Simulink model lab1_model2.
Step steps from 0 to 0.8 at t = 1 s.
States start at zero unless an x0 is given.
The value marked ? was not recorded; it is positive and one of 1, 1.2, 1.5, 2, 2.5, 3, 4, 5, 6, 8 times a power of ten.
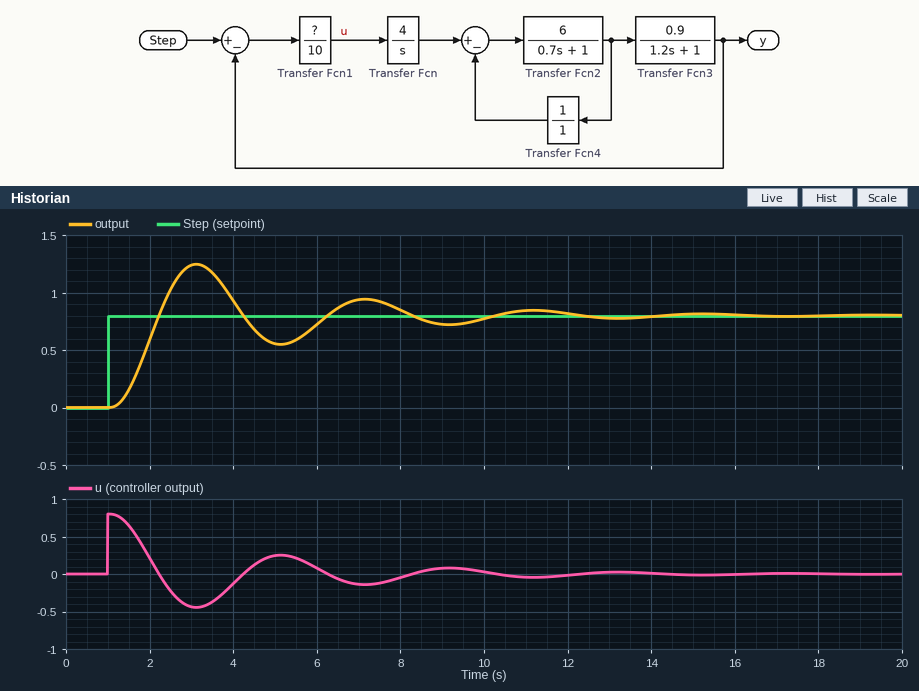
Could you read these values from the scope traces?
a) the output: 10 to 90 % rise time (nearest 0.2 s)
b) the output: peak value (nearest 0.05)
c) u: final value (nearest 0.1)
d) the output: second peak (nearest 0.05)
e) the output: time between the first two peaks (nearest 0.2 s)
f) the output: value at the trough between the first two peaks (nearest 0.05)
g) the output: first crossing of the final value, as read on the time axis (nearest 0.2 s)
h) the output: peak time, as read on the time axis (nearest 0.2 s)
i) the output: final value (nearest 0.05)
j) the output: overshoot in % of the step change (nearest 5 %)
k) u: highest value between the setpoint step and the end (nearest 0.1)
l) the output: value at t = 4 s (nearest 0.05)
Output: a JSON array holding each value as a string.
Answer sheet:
["0.8 s", "1.25", "0.0", "0.95", "4.0 s", "0.55", "2.2 s", "3.2 s", "0.80", "55 %", "0.8", "0.95"]
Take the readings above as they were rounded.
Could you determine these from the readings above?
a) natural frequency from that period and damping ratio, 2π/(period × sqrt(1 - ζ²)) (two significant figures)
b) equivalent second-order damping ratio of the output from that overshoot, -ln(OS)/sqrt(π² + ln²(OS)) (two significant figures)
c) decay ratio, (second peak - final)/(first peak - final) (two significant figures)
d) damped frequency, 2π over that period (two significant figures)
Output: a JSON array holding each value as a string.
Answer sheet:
["1.6 rad/s", "0.19", "0.33", "1.6 rad/s"]
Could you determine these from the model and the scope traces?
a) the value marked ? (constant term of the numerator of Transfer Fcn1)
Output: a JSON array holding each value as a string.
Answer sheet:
["10"]
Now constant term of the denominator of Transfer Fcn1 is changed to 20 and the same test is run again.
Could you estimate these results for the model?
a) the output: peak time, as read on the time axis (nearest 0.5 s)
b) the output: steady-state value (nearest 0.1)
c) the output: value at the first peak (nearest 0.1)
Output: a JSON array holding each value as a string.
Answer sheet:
["4.0 s", "0.8", "1.1"]
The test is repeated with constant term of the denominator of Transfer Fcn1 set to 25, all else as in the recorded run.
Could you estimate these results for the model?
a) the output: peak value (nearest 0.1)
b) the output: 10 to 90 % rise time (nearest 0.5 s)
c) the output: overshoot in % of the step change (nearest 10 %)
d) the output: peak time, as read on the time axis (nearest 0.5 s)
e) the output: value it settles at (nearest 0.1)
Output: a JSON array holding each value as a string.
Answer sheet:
["1.0", "1.5 s", "30 %", "4.5 s", "0.8"]
